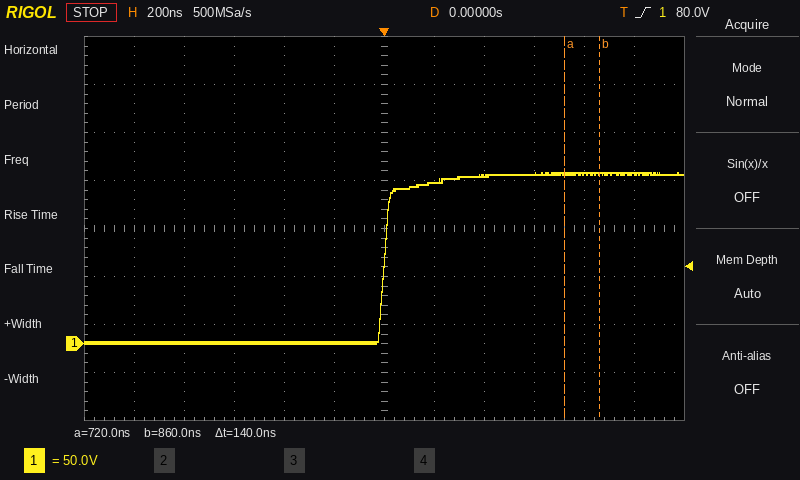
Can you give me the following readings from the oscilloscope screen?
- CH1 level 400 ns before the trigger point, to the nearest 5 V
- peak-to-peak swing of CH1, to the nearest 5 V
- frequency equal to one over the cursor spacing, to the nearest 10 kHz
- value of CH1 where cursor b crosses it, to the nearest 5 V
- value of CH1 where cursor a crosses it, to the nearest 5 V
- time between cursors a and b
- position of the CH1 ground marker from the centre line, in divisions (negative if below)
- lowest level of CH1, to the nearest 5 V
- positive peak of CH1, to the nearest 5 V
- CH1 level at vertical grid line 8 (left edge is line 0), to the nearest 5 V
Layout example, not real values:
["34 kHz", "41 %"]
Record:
["0 V", "180 V", "7.14 MHz", "175 V", "175 V", "140 ns", "-2.4 div", "0 V", "180 V", "175 V"]
